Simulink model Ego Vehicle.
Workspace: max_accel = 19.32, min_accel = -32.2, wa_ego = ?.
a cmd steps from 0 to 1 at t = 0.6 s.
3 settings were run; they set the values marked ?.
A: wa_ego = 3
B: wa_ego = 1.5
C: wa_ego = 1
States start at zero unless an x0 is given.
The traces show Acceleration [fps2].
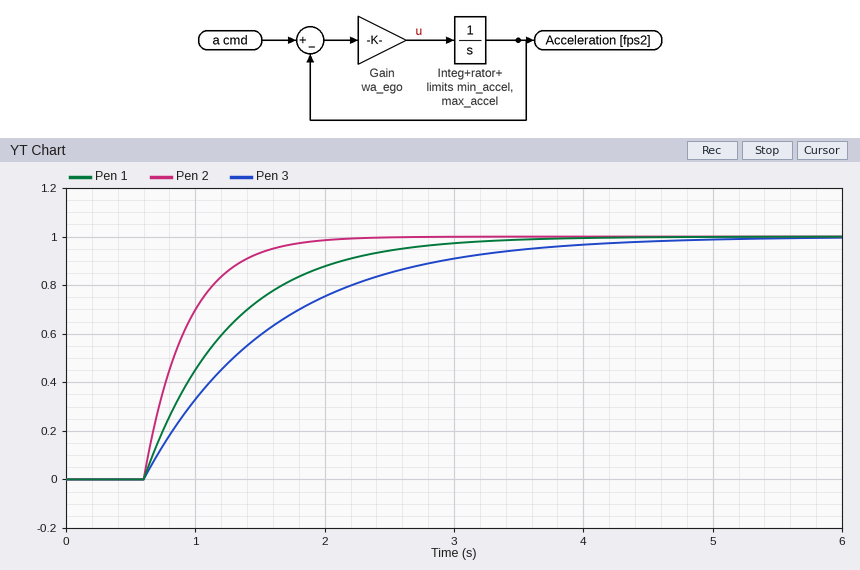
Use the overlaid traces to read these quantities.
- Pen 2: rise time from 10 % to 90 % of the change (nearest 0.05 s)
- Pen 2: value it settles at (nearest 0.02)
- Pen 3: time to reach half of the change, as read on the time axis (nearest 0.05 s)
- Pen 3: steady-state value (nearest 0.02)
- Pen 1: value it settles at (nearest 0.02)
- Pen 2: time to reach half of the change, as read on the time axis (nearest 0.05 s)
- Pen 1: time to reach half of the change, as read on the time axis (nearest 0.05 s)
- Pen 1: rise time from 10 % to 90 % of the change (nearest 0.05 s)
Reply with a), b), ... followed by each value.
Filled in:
a) 0.75 s
b) 1.00
c) 1.30 s
d) 1.00
e) 1.00
f) 0.85 s
g) 1.05 s
h) 1.45 s
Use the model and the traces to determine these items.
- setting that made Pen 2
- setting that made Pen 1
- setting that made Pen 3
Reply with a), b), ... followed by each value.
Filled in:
a) A
b) B
c) C
